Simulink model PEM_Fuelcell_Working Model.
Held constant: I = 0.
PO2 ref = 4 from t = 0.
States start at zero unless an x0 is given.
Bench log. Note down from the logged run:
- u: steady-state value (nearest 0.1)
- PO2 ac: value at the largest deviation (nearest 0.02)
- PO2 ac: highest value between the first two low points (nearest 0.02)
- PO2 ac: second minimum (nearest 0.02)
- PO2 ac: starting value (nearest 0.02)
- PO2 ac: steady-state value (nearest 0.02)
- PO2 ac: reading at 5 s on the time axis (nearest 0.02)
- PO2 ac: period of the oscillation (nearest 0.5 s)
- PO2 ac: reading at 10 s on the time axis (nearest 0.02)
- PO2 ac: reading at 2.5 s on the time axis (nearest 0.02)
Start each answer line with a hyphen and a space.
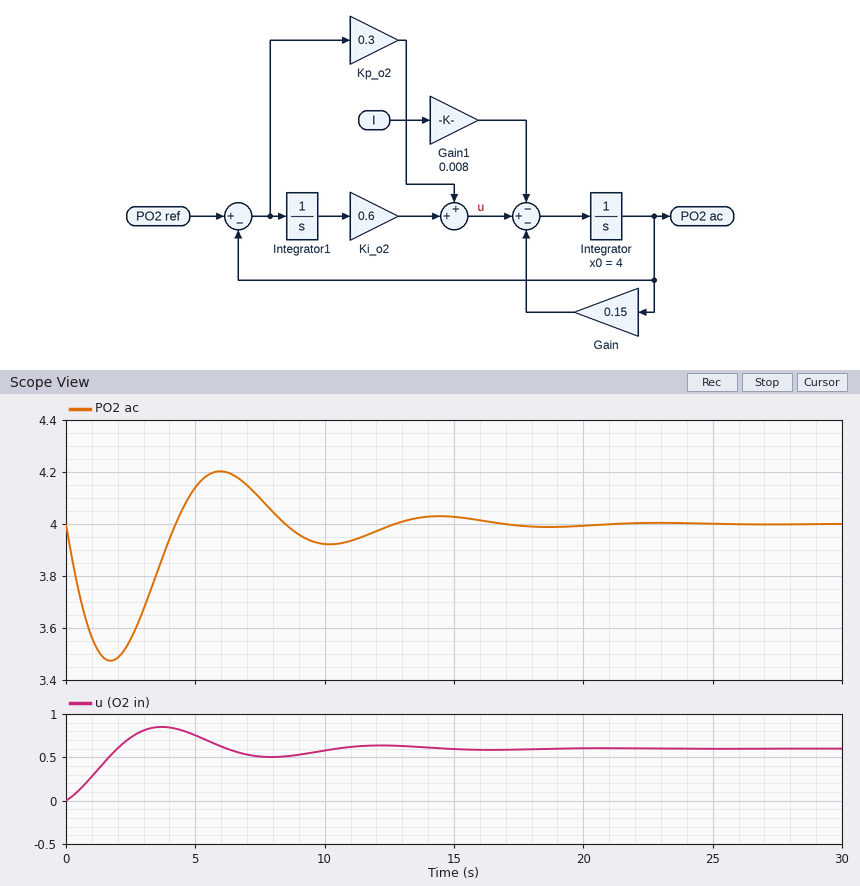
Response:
- 0.6
- 3.48
- 4.20
- 3.92
- 4.00
- 4.00
- 4.14
- 8.5 s
- 3.92
- 3.56
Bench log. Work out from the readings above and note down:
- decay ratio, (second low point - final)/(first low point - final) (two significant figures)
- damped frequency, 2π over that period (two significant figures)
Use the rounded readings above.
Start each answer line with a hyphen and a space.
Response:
- 0.15
- 0.74 rad/s
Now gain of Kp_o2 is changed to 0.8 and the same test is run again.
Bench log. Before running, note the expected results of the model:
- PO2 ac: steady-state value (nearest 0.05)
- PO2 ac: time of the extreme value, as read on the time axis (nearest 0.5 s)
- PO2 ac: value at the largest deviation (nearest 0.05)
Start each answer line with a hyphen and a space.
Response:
- 4.00
- 1.5 s
- 3.60
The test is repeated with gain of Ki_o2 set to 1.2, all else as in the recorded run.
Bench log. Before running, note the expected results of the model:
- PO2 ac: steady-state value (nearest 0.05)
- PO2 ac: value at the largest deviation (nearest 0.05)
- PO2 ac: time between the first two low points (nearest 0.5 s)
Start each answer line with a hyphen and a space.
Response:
- 4.00
- 3.60
- 6.0 s
